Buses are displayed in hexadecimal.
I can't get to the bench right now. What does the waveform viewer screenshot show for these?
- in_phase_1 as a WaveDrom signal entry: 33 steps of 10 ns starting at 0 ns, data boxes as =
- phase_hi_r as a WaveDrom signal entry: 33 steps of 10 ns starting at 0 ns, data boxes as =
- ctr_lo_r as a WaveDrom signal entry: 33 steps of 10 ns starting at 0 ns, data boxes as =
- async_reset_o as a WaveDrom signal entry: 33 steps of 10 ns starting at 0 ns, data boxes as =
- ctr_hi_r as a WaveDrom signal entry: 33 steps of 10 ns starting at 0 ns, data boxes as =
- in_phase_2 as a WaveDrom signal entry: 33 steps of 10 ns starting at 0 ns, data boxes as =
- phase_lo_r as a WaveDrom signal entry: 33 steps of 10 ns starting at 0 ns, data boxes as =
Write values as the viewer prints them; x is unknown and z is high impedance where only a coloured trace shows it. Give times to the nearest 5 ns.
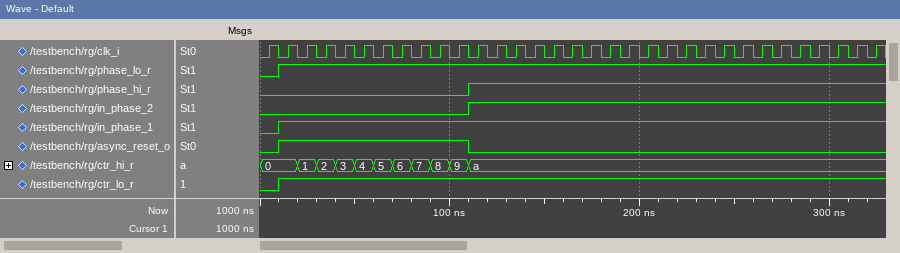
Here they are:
{name: 'in_phase_1', wave: '01...............................'}
{name: 'phase_hi_r', wave: '0..........1.....................'}
{name: 'ctr_lo_r', wave: '01...............................'}
{name: 'async_reset_o', wave: '01.........0.....................'}
{name: 'ctr_hi_r', wave: '=.==========.....................', data: '0 1 2 3 4 5 6 7 8 9 a'}
{name: 'in_phase_2', wave: '0..........1.....................'}
{name: 'phase_lo_r', wave: '01...............................'}
